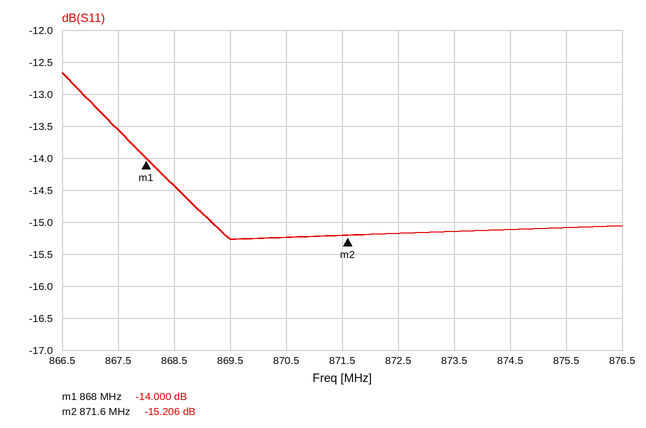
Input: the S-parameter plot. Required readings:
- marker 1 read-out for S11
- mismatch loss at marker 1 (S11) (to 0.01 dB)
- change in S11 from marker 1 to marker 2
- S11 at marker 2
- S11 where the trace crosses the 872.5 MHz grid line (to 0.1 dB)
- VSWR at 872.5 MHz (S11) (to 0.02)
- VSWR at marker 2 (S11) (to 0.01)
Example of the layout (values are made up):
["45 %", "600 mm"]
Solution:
["-14.000 dB", "0.18 dB", "-1.206 dB", "-15.206 dB", "-15.2 dB", "1.42", "1.42"]
